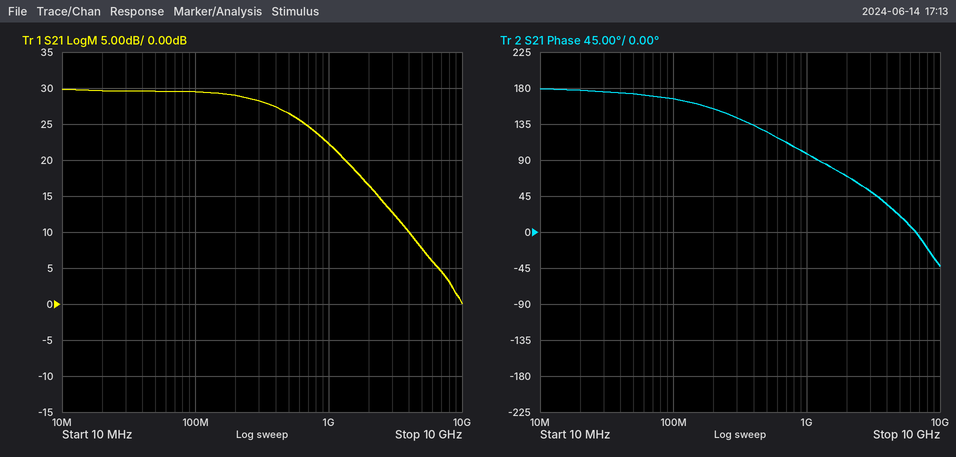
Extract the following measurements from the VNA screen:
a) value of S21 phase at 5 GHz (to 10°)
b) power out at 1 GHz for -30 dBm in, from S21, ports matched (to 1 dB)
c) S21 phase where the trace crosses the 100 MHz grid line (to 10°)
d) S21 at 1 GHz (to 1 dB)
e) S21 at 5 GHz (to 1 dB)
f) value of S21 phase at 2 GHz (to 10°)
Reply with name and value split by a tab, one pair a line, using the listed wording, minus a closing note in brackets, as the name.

value of S21 phase at 5 GHz	20°
power out at 1 GHz for -30 dBm in, from S21, ports matched	-8 dBm
S21 phase where the trace crosses the 100 MHz grid line	170°
S21 at 1 GHz	22 dB
S21 at 5 GHz	8 dB
value of S21 phase at 2 GHz	70°
